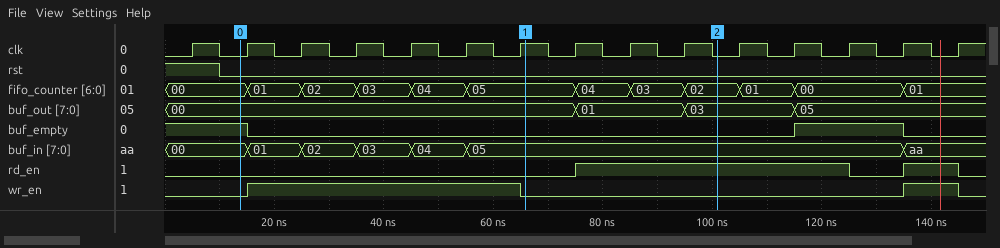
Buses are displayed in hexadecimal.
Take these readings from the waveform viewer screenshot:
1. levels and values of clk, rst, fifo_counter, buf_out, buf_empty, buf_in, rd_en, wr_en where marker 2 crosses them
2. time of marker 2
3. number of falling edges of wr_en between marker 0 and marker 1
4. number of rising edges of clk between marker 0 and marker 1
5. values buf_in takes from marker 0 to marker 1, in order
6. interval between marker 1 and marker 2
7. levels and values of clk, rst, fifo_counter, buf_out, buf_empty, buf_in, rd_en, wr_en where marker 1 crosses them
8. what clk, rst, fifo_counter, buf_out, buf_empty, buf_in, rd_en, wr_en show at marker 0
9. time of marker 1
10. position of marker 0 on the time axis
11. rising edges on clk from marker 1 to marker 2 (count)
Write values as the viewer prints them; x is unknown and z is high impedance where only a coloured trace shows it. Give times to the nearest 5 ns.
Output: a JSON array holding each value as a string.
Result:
["clk=0, rst=0, fifo_counter=02, buf_out=03, buf_empty=0, buf_in=05, rd_en=1, wr_en=0", "100 ns", "1", "6", "00, 01, 02, 03, 04, 05", "35 ns", "clk=1, rst=0, fifo_counter=05, buf_out=00, buf_empty=0, buf_in=05, rd_en=0, wr_en=0", "clk=0, rst=0, fifo_counter=00, buf_out=00, buf_empty=1, buf_in=00, rd_en=0, wr_en=0", "65 ns", "15 ns", "3"]
